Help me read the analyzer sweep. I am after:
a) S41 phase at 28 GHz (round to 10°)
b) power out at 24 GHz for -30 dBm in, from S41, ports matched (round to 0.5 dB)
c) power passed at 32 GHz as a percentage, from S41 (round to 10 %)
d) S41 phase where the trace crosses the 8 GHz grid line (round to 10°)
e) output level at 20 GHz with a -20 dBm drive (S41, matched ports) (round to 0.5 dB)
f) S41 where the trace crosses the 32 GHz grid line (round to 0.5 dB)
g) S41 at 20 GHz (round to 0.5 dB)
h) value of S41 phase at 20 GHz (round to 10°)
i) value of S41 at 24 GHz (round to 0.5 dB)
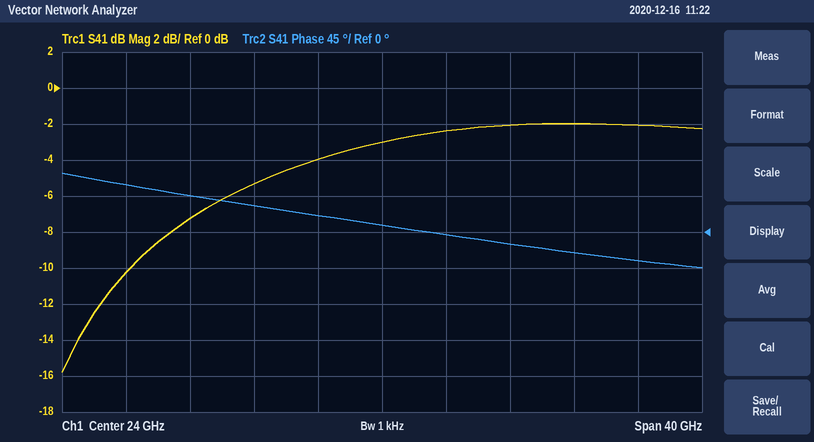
0°
-33.0 dBm
60 %
60°
-24.0 dBm
-2.0 dB
-4.0 dB
20°
-3.0 dB
